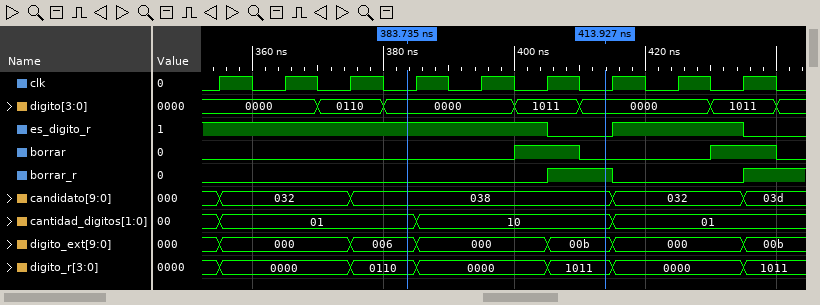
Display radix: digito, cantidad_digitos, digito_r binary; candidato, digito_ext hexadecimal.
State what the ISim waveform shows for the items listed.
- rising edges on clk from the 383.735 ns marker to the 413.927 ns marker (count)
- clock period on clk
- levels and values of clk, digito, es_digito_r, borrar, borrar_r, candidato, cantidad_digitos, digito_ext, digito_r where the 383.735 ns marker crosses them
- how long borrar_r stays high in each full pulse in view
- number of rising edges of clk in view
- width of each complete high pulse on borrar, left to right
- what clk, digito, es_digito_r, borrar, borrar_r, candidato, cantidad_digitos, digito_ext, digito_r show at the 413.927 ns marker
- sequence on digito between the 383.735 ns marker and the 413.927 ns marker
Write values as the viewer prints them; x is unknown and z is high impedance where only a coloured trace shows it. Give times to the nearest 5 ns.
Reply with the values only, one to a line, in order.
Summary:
3
10 ns
clk=0, digito=0000, es_digito_r=1, borrar=0, borrar_r=0, candidato=038, cantidad_digitos=01, digito_ext=006, digito_r=0110
10 ns
9
10 ns, 10 ns
clk=0, digito=0000, es_digito_r=0, borrar=0, borrar_r=1, candidato=038, cantidad_digitos=10, digito_ext=00b, digito_r=1011
0000, 1011, 0000
